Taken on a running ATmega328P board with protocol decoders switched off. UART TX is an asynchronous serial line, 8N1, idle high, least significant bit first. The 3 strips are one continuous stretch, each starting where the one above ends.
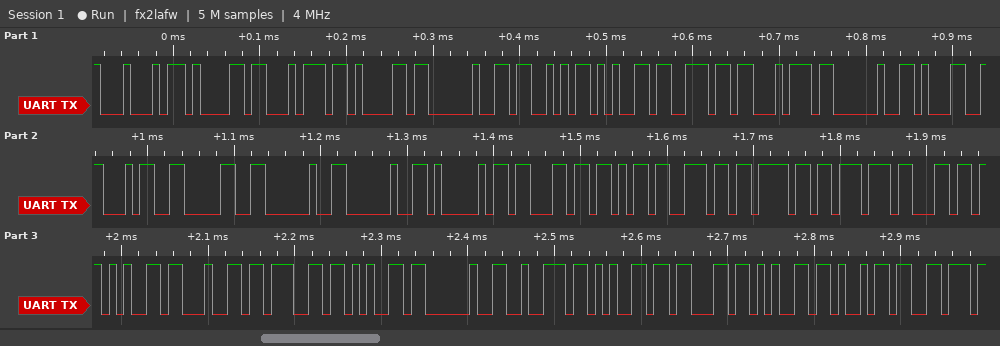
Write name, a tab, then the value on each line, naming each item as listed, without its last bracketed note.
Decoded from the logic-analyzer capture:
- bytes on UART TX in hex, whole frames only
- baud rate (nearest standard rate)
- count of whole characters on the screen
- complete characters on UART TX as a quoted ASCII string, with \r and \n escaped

bytes on UART TX in hex, whole frames only	0x44 0x61 0x74 0x61 0x20 0x53 0x65 0x6E 0x74 0x20 0x31 0x34 0x30 0x20 0x20 0x41 0x63 0x6B 0x6E 0x6F 0x77 0x6C 0x65 0x64 0x67 0x65 0x20 0x72 0x65 0x63 0x65 0x69 0x76
baud rate	115200 baud
count of whole characters on the screen	33
complete characters on UART TX as a quoted ASCII string, with \r and \n escaped	"Data Sent 140  Acknowledge receiv"
